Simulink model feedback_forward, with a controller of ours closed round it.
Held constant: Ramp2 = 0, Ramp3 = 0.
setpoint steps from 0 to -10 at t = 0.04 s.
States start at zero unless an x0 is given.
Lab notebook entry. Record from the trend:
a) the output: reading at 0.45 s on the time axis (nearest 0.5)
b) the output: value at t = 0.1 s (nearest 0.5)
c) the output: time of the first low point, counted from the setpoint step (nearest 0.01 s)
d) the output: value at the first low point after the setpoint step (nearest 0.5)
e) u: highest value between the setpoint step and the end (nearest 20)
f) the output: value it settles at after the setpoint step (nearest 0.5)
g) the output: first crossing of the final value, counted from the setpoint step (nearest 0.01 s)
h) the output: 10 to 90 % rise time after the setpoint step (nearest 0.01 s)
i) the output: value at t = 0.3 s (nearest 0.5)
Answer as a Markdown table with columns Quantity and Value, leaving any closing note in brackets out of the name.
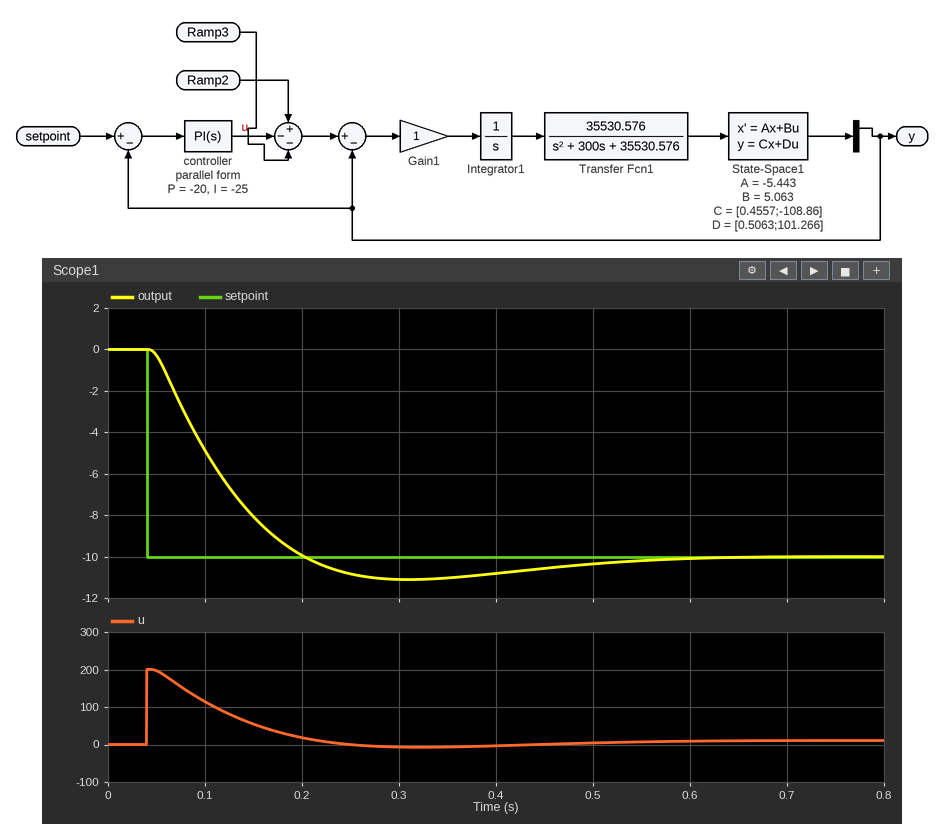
| Quantity | Value |
|---|---|
| the output: reading at 0.45 s on the time axis | -10.5 |
| the output: value at t = 0.1 s | -5.0 |
| the output: time of the first low point, counted from the setpoint step | 0.27 s |
| the output: value at the first low point after the setpoint step | -11.0 |
| u: highest value between the setpoint step and the end | 200 |
| the output: value it settles at after the setpoint step | -10.0 |
| the output: first crossing of the final value, counted from the setpoint step | 0.16 s |
| the output: 10 to 90 % rise time after the setpoint step | 0.11 s |
| the output: value at t = 0.3 s | -11.0 |
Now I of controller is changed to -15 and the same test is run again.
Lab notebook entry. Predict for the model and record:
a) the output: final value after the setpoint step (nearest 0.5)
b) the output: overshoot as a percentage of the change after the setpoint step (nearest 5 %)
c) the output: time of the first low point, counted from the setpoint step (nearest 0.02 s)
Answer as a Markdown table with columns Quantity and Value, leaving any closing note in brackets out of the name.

| Quantity | Value |
|---|---|
| the output: final value after the setpoint step | -10.0 |
| the output: overshoot as a percentage of the change after the setpoint step | 10 % |
| the output: time of the first low point, counted from the setpoint step | 0.28 s |
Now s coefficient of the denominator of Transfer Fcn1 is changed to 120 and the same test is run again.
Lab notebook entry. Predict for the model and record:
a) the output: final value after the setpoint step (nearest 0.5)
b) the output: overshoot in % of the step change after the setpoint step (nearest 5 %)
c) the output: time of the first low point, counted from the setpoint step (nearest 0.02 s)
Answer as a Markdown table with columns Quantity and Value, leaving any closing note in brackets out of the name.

| Quantity | Value |
|---|---|
| the output: final value after the setpoint step | -10.0 |
| the output: overshoot in % of the step change after the setpoint step | 10 % |
| the output: time of the first low point, counted from the setpoint step | 0.28 s |
